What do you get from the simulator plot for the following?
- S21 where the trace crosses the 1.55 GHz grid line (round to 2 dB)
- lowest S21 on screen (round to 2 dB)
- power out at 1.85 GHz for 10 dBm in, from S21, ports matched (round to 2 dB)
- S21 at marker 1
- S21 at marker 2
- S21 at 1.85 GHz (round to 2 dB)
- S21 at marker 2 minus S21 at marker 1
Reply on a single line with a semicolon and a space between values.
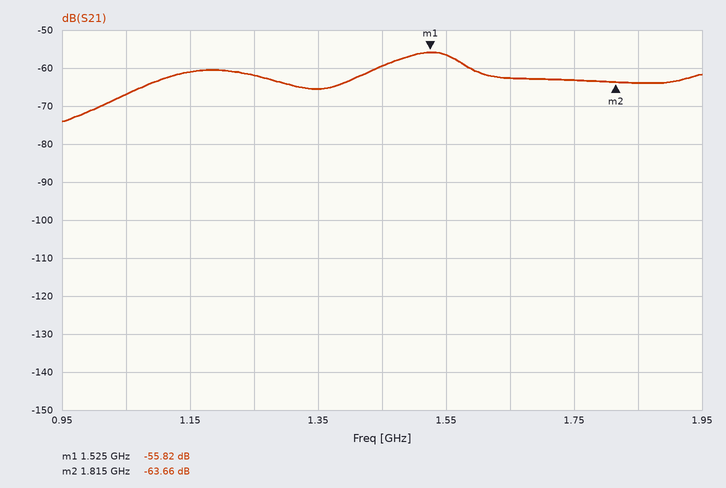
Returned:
-56 dB; -74 dB; -54 dBm; -55.82 dB; -63.66 dB; -64 dB; -7.84 dB
